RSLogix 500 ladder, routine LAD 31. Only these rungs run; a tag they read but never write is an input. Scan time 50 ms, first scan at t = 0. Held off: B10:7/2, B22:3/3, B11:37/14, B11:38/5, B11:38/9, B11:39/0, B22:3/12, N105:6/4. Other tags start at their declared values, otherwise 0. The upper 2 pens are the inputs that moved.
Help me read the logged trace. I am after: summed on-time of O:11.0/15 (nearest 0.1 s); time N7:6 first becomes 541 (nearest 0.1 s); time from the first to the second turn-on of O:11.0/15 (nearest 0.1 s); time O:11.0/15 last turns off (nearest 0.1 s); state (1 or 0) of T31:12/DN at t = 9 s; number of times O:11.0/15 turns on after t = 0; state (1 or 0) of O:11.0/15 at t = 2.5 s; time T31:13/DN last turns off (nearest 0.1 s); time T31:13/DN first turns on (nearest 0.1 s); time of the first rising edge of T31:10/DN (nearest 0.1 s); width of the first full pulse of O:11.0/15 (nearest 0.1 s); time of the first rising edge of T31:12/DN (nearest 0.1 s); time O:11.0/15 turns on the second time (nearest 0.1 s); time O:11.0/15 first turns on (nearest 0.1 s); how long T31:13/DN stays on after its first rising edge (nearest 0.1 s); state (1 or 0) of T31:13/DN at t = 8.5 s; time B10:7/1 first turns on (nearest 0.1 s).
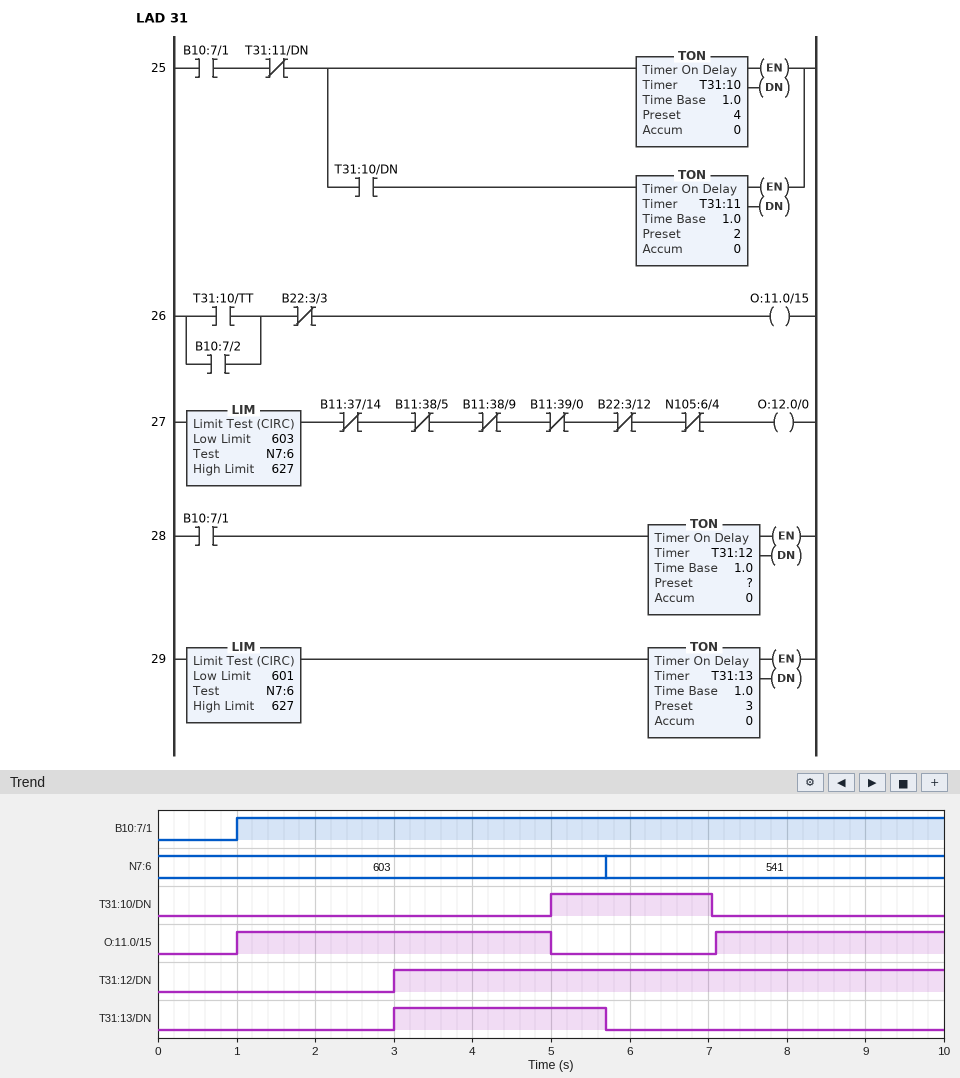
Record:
6.9 s
5.7 s
6.1 s
5.0 s
1
2
1
5.7 s
3.0 s
5.0 s
4.0 s
3.0 s
7.1 s
1.0 s
2.7 s
0
1.0 s
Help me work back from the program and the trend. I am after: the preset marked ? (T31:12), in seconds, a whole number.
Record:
2 s
